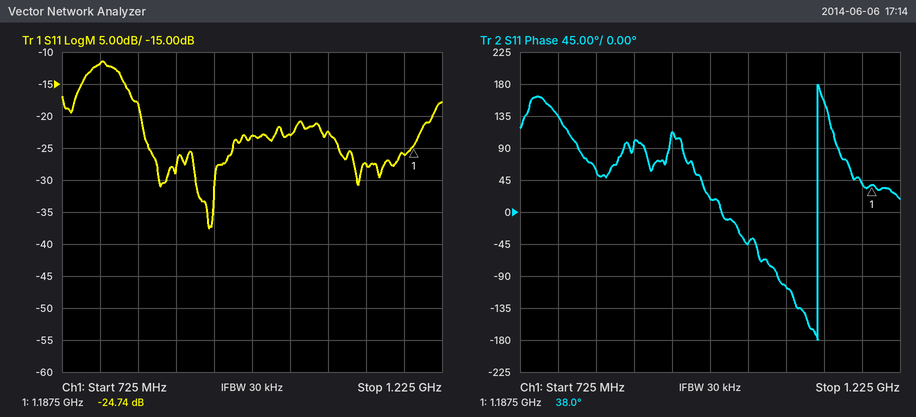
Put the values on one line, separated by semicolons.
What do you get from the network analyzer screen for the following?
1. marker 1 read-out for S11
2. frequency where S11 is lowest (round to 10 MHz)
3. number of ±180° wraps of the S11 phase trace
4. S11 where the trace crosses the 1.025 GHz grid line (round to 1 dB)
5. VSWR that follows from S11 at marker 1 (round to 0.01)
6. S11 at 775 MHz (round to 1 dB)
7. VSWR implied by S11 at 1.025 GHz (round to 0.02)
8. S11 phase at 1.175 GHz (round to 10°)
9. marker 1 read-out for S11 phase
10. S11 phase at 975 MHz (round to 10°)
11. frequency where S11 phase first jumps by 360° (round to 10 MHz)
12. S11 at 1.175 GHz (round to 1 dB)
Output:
-24.74 dB; 920 MHz; 1; -23 dB; 1.12; -12 dB; 1.16; 40°; 38.0°; 20°; 1.12 GHz; -26 dB
